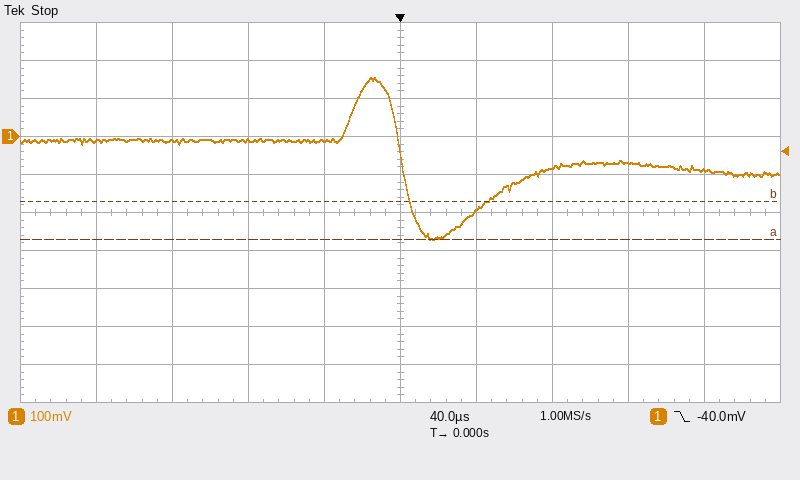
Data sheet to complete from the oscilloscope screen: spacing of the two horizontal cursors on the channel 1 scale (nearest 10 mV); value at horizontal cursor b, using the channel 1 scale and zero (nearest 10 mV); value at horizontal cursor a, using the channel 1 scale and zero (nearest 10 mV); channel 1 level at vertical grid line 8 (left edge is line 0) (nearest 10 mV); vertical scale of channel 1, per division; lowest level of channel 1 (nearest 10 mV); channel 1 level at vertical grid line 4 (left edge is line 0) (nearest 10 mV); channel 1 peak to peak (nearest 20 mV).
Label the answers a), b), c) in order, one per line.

a) 100 mV
b) -170 mV
c) -270 mV
d) -70 mV
e) 100 mV
f) -270 mV
g) -10 mV
h) 420 mV
